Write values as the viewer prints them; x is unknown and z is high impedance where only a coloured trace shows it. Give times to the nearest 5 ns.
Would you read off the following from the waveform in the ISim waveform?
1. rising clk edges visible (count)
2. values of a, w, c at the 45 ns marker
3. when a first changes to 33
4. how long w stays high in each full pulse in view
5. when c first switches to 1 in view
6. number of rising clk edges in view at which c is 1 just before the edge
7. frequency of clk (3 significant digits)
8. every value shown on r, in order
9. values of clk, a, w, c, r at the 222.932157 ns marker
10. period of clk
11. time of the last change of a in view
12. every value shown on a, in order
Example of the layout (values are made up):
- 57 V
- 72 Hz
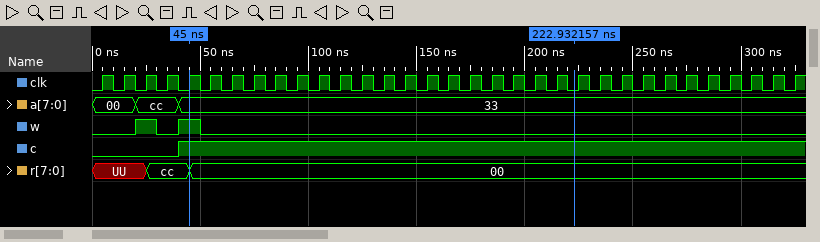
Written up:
- 33
- a=33, w=1, c=1
- 40 ns
- 10 ns, 10 ns
- 40 ns
- 29
- 100 MHz
- UU, cc, 00
- clk=0, a=33, w=0, c=1, r=00
- 10 ns
- 40 ns
- 00, cc, 33
